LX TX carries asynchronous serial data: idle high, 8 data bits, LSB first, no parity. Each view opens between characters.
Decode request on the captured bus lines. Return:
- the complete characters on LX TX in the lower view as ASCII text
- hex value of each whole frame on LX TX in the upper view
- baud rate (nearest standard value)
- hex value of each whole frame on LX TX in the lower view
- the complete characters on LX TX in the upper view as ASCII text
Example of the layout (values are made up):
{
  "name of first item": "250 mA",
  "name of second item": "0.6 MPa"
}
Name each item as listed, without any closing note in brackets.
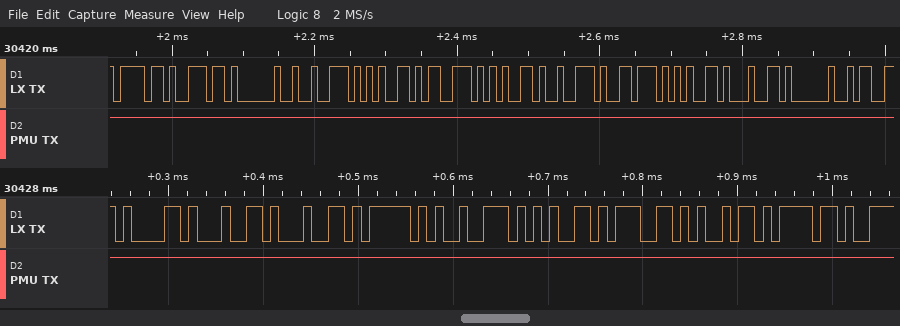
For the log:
{
  "the complete characters on LX TX in the lower view as ASCII text": "\"add_regio\"",
  "hex value of each whole frame on LX TX in the upper view": "6F, 6E, 20, 72, 65, 73, 65, 72, 76, 65, 64, 20",
  "baud rate": "115200 baud",
  "hex value of each whole frame on LX TX in the lower view": "61, 64, 64, 5F, 72, 65, 67, 69, 6F",
  "the complete characters on LX TX in the upper view as ASCII text": "\"on reserved \""
}
